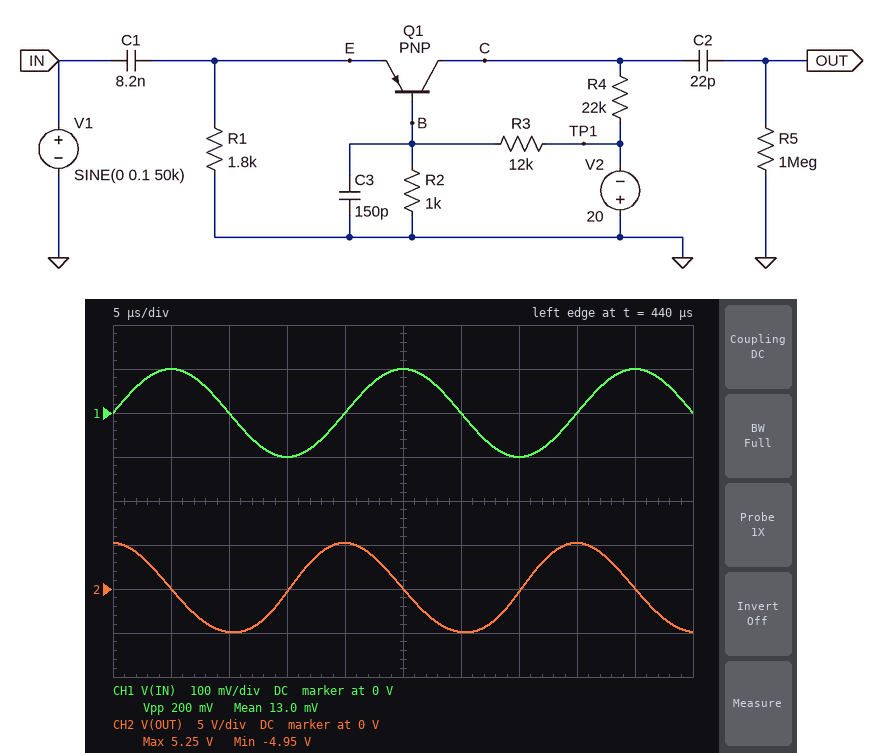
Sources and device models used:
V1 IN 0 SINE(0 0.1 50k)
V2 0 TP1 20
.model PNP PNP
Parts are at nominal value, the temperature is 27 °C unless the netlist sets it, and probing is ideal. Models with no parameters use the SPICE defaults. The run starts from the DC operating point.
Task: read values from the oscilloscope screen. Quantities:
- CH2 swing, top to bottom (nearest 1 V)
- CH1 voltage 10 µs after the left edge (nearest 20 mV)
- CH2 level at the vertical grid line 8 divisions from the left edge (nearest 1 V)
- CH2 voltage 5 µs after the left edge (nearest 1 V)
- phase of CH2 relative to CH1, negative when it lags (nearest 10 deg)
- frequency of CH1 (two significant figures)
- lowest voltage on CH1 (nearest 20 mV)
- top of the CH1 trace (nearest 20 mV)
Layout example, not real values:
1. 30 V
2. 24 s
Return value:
1. 10 V
2. 0 V
3. 5 V
4. 0 V
5. 90 deg
6. 50 kHz
7. -100 mV
8. 100 mV
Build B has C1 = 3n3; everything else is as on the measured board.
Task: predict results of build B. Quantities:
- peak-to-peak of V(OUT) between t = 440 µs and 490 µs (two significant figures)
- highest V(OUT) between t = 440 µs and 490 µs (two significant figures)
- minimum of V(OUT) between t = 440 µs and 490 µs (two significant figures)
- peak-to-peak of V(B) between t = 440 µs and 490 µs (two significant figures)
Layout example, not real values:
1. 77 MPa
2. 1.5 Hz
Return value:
1. 4.2 V
2. 2.1 V
3. -2.1 V
4. 1.8 mV
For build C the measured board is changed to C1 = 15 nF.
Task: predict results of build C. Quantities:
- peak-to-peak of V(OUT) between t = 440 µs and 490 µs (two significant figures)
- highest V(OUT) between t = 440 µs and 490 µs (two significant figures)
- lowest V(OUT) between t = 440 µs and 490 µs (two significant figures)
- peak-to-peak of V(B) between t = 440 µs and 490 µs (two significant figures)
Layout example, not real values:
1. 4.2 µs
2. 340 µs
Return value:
1. 17 V
2. 9.6 V
3. -7.5 V
4. 7.5 mV
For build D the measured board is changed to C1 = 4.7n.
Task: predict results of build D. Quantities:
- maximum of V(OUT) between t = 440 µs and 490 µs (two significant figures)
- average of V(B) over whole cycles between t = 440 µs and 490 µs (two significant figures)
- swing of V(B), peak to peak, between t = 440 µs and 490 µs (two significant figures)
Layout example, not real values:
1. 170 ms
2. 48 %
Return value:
1. 3.0 V
2. -1.5 V
3. 2.6 mV
